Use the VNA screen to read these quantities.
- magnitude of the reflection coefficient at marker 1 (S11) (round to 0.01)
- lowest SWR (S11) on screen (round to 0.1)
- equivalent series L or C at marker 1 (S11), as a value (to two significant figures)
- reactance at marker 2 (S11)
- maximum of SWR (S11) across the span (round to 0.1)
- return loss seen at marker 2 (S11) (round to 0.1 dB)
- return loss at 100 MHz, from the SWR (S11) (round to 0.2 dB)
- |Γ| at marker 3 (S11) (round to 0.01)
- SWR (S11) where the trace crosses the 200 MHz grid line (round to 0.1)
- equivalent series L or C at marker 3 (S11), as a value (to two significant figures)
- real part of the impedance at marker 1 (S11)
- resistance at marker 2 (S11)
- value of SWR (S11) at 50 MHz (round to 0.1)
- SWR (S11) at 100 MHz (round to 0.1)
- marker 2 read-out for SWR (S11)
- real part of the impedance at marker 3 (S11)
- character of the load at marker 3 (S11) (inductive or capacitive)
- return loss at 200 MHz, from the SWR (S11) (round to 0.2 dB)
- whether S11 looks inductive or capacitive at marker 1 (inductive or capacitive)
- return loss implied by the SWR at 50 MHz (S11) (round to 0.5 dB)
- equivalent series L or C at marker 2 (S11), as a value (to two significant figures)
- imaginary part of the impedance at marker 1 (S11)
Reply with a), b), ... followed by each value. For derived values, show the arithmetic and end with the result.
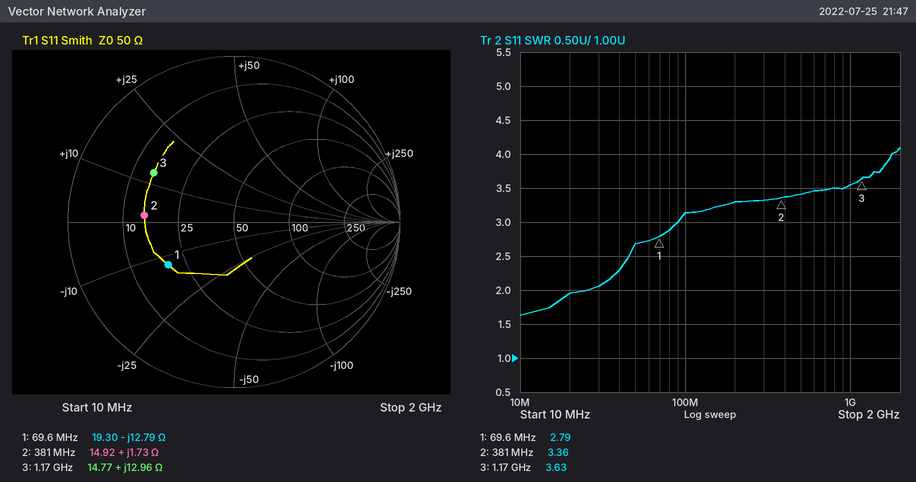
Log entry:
a) 0.47
b) 1.6
c) C = 1/(2π × 69.6 MHz × 12.79 Ω) ≈ 179 pF, so 180 pF to two significant figures
d) +1.73 Ω
e) 4.1
f) 5.3 dB
g) −20 log10((3.1 − 1)/(3.1 + 1)) ≈ 5.8 dB
h) 0.57
i) 3.3
j) L = 12.96 Ω/(2π × 1.17 GHz) ≈ 1.8 nH
k) 19.30 Ω
l) 14.92 Ω
m) 2.7
n) 3.1
o) 3.36
p) 14.77 Ω
q) inductive
r) −20 log10((3.3 − 1)/(3.3 + 1)) ≈ 5.4 dB
s) capacitive
t) −20 log10((2.7 − 1)/(2.7 + 1)) ≈ 6.76 dB, so 7.0 dB to the nearest 0.5 dB
u) L = 1.73 Ω/(2π × 381 MHz) ≈ 723 pH, so 720 pH to two significant figures
v) -12.79 Ω
